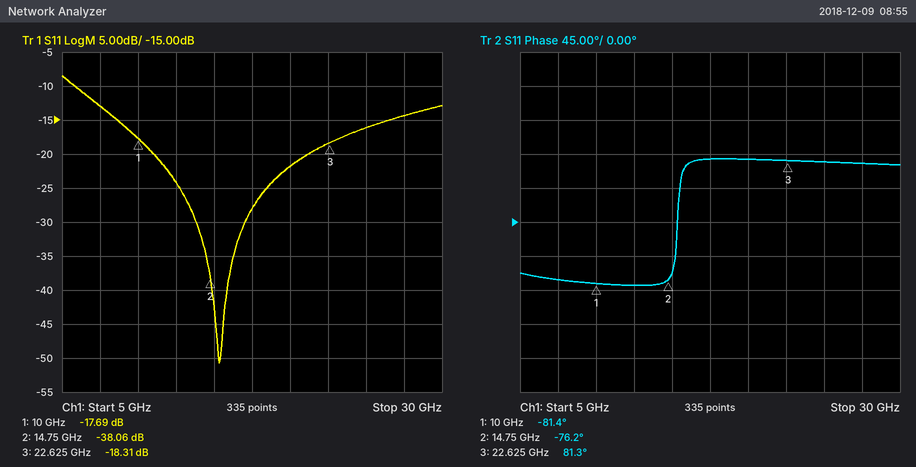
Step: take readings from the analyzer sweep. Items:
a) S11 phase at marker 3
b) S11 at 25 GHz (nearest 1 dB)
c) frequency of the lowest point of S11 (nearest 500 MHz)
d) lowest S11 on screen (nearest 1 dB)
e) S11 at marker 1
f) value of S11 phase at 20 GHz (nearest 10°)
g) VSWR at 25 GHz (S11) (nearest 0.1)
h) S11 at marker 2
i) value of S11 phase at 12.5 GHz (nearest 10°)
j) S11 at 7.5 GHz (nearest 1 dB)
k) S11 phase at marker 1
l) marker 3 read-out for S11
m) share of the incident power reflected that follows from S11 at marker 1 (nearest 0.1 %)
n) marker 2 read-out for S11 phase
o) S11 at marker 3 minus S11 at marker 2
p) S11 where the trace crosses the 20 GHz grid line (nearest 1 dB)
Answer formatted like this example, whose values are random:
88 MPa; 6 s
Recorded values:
81.3°; -16 dB; 15.5 GHz; -51 dB; -17.69 dB; 80°; 1.4; -38.06 dB; -80°; -13 dB; -81.4°; -18.31 dB; 1.7 %; -76.2°; 19.75 dB; -22 dB
